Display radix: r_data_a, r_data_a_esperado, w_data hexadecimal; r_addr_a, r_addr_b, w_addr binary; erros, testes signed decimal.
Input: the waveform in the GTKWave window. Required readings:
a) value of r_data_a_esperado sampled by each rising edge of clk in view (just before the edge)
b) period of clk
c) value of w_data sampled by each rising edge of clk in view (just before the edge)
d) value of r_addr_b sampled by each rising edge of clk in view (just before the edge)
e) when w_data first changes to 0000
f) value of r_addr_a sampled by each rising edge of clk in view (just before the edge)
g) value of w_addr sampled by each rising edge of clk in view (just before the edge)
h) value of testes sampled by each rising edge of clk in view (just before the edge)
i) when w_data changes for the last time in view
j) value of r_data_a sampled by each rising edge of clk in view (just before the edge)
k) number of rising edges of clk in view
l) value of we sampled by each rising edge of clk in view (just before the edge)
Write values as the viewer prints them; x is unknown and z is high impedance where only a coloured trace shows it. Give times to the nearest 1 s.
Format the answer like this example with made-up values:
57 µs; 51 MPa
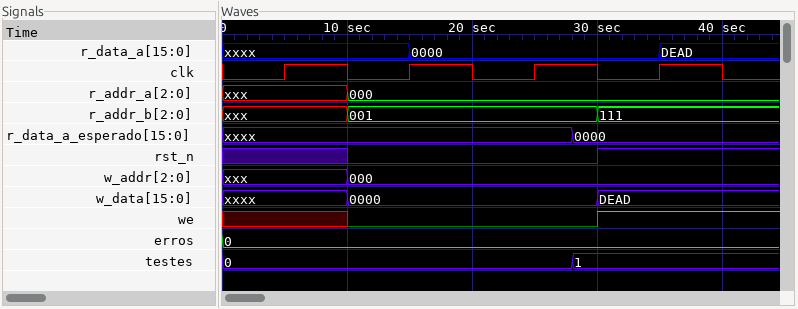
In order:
xxxx, xxxx, xxxx, 0000; 10 s; xxxx, 0000, 0000, DEAD; xxx, 001, 001, 111; 10 s; xxx, 000, 000, 000; xxx, 000, 000, 000; 0, 0, 0, 1; 30 s; xxxx, xxxx, 0000, 0000; 4; x 0 0 1
